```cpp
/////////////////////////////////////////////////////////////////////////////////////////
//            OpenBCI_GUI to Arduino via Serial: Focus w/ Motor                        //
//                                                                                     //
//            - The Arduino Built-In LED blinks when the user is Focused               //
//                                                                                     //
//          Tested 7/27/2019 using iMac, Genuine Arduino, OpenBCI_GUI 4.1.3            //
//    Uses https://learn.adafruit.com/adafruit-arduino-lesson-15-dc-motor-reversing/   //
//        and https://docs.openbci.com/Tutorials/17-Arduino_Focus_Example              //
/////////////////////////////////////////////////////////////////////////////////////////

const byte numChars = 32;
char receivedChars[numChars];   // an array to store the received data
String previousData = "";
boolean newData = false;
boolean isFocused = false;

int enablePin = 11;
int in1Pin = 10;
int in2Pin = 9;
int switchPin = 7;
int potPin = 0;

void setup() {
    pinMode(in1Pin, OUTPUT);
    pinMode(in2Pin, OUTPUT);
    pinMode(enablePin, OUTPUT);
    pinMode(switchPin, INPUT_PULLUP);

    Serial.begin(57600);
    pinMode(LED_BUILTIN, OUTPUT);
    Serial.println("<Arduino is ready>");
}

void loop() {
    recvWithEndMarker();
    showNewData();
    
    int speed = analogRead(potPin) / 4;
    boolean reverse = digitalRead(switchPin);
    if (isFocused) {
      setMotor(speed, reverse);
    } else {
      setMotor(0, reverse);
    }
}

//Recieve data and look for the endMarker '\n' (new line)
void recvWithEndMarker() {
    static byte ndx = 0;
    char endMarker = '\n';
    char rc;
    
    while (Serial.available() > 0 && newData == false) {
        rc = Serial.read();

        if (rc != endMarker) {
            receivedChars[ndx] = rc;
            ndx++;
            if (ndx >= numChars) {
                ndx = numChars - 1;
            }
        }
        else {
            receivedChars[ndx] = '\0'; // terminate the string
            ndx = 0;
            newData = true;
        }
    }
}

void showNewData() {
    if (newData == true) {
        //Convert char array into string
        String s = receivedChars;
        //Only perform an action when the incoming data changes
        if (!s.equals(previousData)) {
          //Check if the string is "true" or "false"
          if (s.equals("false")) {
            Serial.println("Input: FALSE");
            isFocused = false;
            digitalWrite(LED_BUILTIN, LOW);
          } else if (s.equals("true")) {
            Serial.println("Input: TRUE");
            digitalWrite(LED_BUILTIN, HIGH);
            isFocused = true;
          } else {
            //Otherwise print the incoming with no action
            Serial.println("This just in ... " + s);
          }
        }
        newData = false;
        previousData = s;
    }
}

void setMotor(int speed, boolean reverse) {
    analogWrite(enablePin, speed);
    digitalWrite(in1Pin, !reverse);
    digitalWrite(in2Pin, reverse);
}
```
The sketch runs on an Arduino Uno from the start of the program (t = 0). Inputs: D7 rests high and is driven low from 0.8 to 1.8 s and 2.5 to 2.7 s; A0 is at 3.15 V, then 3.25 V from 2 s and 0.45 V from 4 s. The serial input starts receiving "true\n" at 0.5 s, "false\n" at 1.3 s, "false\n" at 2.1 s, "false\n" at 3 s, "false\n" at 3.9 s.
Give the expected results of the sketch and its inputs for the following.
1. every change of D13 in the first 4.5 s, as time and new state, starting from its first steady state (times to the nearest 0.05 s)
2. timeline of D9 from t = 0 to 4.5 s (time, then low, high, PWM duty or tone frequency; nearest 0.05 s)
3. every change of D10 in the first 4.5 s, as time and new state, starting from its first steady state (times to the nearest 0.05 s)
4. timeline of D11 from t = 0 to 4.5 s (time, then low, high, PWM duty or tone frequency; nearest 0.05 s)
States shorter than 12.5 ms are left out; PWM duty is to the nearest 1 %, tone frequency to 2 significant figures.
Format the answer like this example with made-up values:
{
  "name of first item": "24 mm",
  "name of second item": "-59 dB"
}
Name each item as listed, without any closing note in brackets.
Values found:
{
  "every change of D13 in the first 4.5 s, as time and new state, starting from its first steady state": "0 s low; 0.5 s high; 1.3 s low",
  "timeline of D9 from t = 0 to 4.5 s": "0 s high; 0.8 s low; 1.8 s high; 2.5 s low; 2.7 s high",
  "every change of D10 in the first 4.5 s, as time and new state, starting from its first steady state": "0 s low; 0.8 s high; 1.8 s low; 2.5 s high; 2.7 s low",
  "timeline of D11 from t = 0 to 4.5 s": "0 s low; 0.5 s PWM 63 %; 1.3 s low"
}
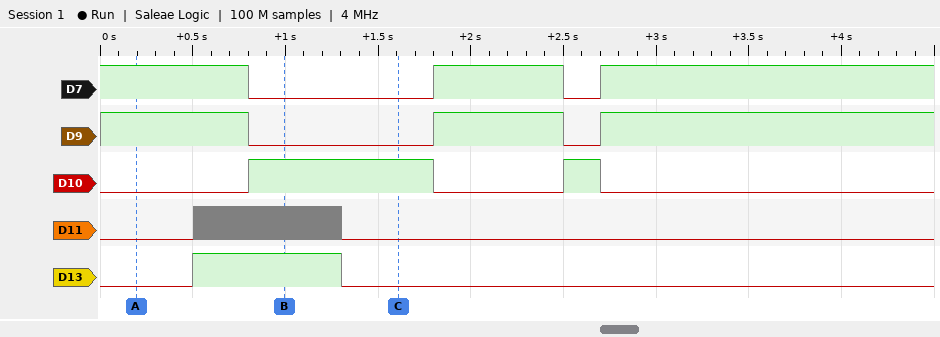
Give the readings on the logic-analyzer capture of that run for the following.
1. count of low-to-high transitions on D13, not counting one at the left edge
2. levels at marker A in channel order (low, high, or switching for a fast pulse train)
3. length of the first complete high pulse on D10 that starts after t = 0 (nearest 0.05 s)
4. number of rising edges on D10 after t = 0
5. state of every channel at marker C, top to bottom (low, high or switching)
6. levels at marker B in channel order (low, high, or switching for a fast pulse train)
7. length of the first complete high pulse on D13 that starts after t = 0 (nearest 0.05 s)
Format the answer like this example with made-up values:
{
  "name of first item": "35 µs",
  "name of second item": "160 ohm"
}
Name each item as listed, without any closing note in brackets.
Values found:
{
  "count of low-to-high transitions on D13, not counting one at the left edge": "1",
  "levels at marker A in channel order": "D7 high, D9 high, D10 low, D11 low, D13 low",
  "length of the first complete high pulse on D10 that starts after t = 0": "1.00 s",
  "number of rising edges on D10 after t = 0": "2",
  "state of every channel at marker C, top to bottom": "D7 low, D9 low, D10 high, D11 low, D13 low",
  "levels at marker B in channel order": "D7 low, D9 low, D10 high, D11 switching, D13 high",
  "length of the first complete high pulse on D13 that starts after t = 0": "0.80 s"
}
